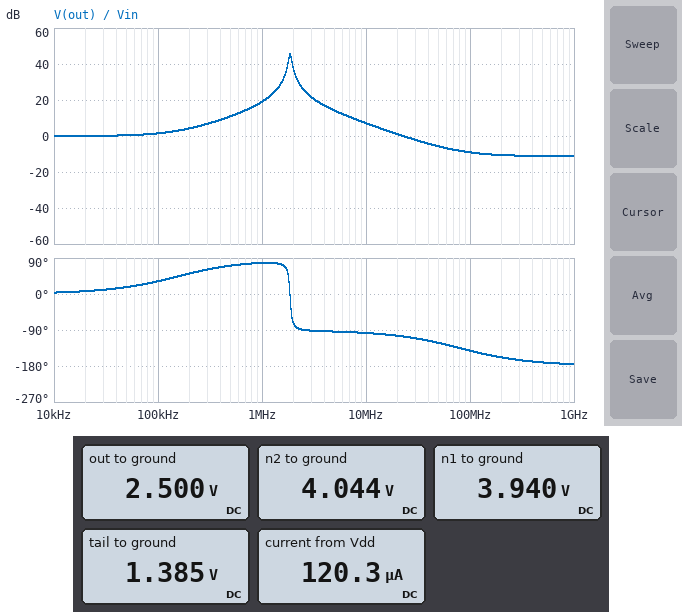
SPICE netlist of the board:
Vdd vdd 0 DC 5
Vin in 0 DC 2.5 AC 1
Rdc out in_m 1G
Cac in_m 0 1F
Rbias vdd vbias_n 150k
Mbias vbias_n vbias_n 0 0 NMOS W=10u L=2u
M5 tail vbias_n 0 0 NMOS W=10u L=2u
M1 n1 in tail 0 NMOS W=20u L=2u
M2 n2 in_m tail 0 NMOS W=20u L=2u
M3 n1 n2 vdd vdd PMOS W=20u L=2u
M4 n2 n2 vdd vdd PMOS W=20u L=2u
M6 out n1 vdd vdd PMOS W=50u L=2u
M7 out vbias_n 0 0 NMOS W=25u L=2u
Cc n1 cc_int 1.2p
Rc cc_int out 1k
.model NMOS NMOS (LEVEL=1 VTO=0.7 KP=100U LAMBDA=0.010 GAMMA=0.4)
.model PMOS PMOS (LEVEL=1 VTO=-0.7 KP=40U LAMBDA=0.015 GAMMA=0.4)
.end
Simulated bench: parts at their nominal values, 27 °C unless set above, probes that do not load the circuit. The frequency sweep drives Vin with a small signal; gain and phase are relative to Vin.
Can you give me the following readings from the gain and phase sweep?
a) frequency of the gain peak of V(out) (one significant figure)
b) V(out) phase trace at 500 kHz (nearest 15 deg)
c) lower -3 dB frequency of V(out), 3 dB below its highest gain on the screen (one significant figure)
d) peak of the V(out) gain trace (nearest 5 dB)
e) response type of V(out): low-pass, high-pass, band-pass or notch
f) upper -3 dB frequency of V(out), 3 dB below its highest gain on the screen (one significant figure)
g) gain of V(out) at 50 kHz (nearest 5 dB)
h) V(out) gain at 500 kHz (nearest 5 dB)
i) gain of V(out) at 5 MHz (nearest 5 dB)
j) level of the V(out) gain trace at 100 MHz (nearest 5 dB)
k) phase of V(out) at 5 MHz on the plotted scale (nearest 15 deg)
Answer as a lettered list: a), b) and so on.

a) 2 MHz
b) 75 deg
c) 2 MHz
d) 45 dB
e) band-pass
f) 2 MHz
g) 0 dB
h) 10 dB
i) 15 dB
j) -10 dB
k) -90 deg
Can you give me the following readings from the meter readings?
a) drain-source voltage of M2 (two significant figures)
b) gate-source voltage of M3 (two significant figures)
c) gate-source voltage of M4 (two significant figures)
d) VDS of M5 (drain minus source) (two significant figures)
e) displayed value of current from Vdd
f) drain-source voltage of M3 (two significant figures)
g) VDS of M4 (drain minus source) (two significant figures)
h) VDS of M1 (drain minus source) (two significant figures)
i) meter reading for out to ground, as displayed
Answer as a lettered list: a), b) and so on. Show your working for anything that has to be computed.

a) 4.044 V - 1.385 V = 2.7 V
b) 4.044 V - 5 V = -960 mV
c) 4.044 V - 5 V = -960 mV
d) 1.385 V = 1.4 V
e) 120.3 µA
f) 3.94 V - 5 V = -1.1 V
g) 4.044 V - 5 V = -960 mV
h) 3.94 V - 1.385 V = 2.6 V
i) 2.500 V
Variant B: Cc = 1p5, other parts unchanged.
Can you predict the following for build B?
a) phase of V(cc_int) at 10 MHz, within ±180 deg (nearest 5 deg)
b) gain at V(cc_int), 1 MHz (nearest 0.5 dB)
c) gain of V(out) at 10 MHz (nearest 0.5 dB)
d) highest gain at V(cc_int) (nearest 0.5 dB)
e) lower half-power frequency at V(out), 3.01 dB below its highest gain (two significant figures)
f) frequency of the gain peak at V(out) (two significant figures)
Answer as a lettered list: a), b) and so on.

a) -105 deg
b) 20.0 dB
c) 5.0 dB
d) 43.5 dB
e) 1.6 MHz
f) 1.7 MHz
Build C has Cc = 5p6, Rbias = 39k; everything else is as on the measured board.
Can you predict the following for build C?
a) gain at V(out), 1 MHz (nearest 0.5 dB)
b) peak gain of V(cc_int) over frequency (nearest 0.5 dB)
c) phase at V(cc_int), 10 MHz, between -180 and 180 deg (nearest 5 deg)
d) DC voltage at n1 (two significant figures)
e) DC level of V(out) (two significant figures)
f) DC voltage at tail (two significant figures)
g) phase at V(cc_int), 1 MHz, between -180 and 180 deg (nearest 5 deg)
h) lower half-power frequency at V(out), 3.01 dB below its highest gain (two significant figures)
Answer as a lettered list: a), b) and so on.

a) 26.5 dB
b) 36.0 dB
c) -115 deg
d) 3.6 V
e) 2.5 V
f) 1.3 V
g) 60 deg
h) 1.1 MHz
